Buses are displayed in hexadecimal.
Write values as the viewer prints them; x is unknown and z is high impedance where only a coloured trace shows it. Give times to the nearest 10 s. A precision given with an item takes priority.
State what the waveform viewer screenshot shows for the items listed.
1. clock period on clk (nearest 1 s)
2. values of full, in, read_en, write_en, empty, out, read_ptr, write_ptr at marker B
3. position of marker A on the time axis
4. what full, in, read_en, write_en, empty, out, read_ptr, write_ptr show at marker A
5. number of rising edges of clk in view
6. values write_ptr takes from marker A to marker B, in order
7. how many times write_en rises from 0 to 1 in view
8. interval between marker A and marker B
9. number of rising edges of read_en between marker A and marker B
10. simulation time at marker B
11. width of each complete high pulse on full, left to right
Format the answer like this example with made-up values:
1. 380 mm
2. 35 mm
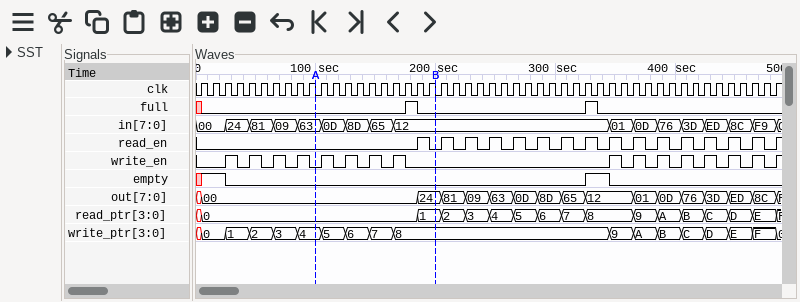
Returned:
1. 10 s
2. full=0, in=12, read_en=0, write_en=0, empty=0, out=24, read_ptr=1, write_ptr=8
3. 100 s
4. full=0, in=63, read_en=0, write_en=0, empty=0, out=00, read_ptr=0, write_ptr=4
5. 49
6. 4, 5, 6, 7, 8
7. 16
8. 100 s
9. 1
10. 200 s
11. 10 s, 10 s
